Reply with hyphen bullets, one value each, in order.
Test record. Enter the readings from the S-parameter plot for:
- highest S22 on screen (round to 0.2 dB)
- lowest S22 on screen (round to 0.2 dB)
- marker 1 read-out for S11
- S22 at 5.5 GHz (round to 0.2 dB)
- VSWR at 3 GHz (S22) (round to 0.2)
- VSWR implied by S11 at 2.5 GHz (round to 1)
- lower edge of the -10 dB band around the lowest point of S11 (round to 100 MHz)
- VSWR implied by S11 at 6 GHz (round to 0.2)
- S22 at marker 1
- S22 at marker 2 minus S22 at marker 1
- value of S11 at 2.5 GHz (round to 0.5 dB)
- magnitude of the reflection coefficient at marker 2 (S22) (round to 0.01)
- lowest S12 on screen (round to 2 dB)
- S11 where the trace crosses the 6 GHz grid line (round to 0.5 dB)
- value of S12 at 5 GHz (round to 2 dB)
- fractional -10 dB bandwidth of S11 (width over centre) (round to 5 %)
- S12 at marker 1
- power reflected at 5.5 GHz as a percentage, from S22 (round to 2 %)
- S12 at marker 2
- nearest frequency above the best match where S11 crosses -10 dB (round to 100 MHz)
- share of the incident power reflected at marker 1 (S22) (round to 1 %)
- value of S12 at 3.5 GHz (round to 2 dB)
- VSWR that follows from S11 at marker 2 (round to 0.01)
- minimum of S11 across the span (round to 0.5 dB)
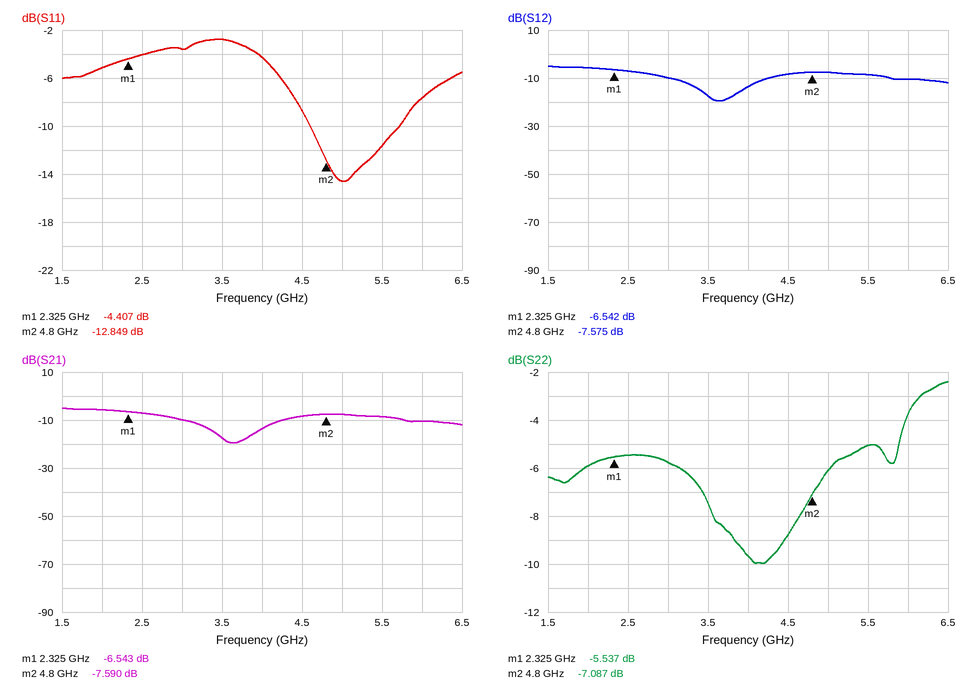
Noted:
- -2.4 dB
- -10.0 dB
- -4.407 dB
- -5.0 dB
- 3.2
- 4
- 4.6 GHz
- 2.4
- -5.537 dB
- -1.550 dB
- -4.0 dB
- 0.44
- -20 dB
- -7.5 dB
- -8 dB
- 20 %
- -6.542 dB
- 32 %
- -7.575 dB
- 5.7 GHz
- 28 %
- -18 dB
- 1.59
- -14.5 dB
